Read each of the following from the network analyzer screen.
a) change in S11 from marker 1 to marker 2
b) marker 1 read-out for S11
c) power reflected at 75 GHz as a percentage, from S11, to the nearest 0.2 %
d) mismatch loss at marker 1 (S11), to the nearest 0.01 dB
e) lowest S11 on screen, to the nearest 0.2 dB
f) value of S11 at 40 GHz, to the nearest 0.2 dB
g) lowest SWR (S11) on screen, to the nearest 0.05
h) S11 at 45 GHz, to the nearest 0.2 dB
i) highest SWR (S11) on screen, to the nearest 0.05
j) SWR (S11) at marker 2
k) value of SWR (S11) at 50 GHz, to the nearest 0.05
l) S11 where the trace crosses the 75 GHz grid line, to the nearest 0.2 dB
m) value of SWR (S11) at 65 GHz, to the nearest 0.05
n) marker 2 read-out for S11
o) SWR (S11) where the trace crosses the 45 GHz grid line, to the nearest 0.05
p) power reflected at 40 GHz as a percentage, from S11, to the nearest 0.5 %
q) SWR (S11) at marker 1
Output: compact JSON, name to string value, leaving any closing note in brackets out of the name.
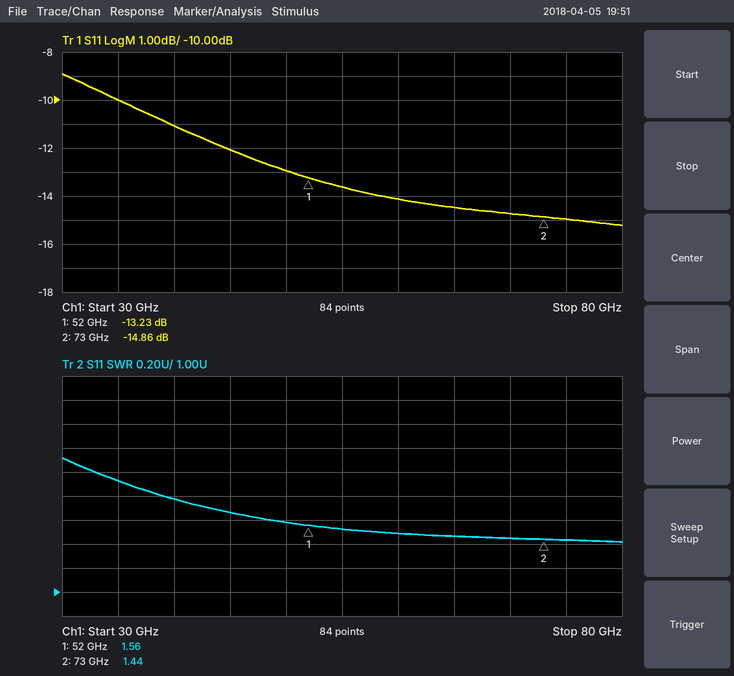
{"change in S11 from marker 1 to marker 2": "-1.63 dB", "marker 1 read-out for S11": "-13.23 dB", "power reflected at 75 GHz as a percentage, from S11, to the nearest 0.2 %": "3.2 %", "mismatch loss at marker 1 (S11), to the nearest 0.01 dB": "0.21 dB", "lowest S11 on screen, to the nearest 0.2 dB": "-15.2 dB", "value of S11 at 40 GHz, to the nearest 0.2 dB": "-11.0 dB", "lowest SWR (S11) on screen, to the nearest 0.05": "1.40", "S11 at 45 GHz, to the nearest 0.2 dB": "-12.0 dB", "highest SWR (S11) on screen, to the nearest 0.05": "2.10", "SWR (S11) at marker 2": "1.44", "value of SWR (S11) at 50 GHz, to the nearest 0.05": "1.60", "S11 where the trace crosses the 75 GHz grid line, to the nearest 0.2 dB": "-15.0 dB", "value of SWR (S11) at 65 GHz, to the nearest 0.05": "1.45", "marker 2 read-out for S11": "-14.86 dB", "SWR (S11) where the trace crosses the 45 GHz grid line, to the nearest 0.05": "1.65", "power reflected at 40 GHz as a percentage, from S11, to the nearest 0.5 %": "8.0 %", "SWR (S11) at marker 1": "1.56"}
